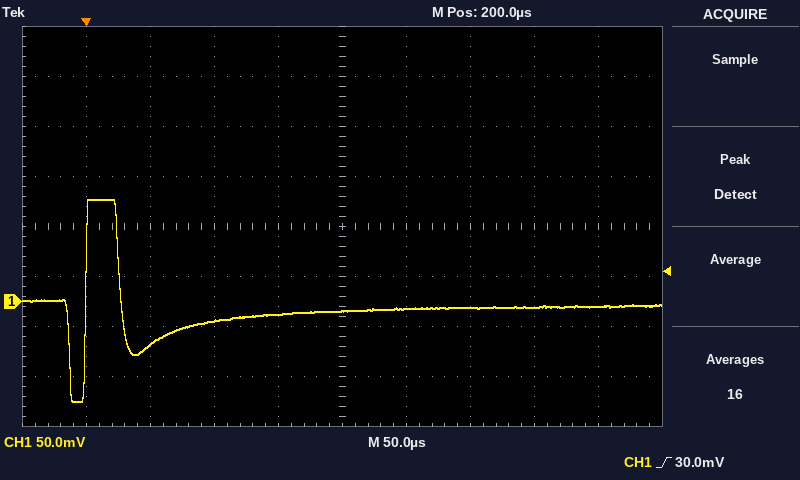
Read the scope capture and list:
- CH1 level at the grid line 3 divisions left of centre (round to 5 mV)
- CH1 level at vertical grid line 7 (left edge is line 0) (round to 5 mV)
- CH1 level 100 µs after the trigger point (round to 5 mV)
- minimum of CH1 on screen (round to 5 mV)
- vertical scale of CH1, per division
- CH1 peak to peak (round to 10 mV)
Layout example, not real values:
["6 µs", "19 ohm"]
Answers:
["-45 mV", "-5 mV", "-20 mV", "-100 mV", "50 mV", "200 mV"]
